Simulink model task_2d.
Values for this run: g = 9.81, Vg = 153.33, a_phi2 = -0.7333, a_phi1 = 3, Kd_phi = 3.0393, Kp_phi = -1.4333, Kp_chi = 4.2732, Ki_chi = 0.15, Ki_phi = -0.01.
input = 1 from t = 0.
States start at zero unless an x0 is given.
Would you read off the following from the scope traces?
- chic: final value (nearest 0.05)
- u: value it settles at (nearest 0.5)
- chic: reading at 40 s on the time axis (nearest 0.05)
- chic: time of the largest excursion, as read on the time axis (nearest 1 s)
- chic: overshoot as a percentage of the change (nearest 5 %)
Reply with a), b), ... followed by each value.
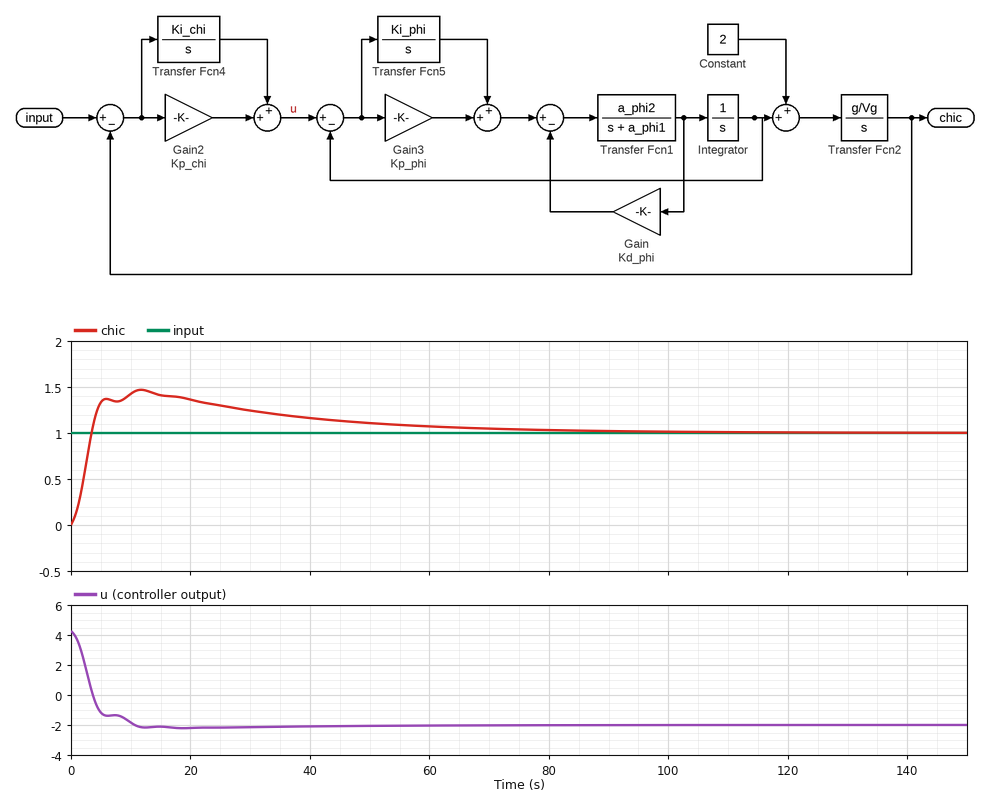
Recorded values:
a) 1.00
b) -2.0
c) 1.15
d) 12 s
e) 45 %
